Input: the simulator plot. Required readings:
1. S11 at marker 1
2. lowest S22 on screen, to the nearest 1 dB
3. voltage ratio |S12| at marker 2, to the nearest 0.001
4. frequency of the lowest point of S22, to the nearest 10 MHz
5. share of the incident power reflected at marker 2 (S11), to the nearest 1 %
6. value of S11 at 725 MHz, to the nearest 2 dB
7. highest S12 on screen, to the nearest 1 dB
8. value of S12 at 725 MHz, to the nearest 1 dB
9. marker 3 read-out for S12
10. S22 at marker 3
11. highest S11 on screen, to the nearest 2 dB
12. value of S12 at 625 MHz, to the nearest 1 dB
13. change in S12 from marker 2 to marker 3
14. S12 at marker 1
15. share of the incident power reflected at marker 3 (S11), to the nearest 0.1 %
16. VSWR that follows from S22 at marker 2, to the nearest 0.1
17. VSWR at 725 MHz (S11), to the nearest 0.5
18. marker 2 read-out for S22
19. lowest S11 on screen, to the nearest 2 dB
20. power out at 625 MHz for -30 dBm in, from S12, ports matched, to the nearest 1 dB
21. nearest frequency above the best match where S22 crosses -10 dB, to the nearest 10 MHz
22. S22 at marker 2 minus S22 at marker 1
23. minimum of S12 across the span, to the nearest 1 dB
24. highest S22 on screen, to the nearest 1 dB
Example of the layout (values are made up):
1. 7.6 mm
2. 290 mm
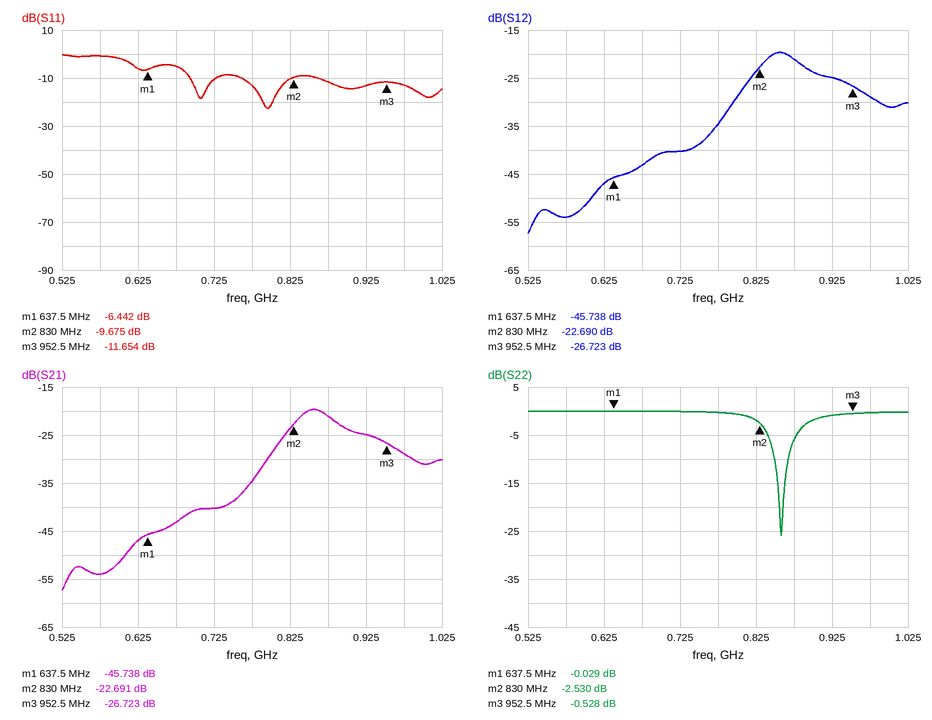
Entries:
1. -6.442 dB
2. -26 dB
3. 0.073
4. 860 MHz
5. 11 %
6. -10 dB
7. -20 dB
8. -40 dB
9. -26.723 dB
10. -0.528 dB
11. 0 dB
12. -47 dB
13. -4.033 dB
14. -45.738 dB
15. 6.8 %
16. 6.9
17. 2.0
18. -2.530 dB
19. -22 dB
20. -77 dBm
21. 870 MHz
22. -2.501 dB
23. -57 dB
24. 0 dB
